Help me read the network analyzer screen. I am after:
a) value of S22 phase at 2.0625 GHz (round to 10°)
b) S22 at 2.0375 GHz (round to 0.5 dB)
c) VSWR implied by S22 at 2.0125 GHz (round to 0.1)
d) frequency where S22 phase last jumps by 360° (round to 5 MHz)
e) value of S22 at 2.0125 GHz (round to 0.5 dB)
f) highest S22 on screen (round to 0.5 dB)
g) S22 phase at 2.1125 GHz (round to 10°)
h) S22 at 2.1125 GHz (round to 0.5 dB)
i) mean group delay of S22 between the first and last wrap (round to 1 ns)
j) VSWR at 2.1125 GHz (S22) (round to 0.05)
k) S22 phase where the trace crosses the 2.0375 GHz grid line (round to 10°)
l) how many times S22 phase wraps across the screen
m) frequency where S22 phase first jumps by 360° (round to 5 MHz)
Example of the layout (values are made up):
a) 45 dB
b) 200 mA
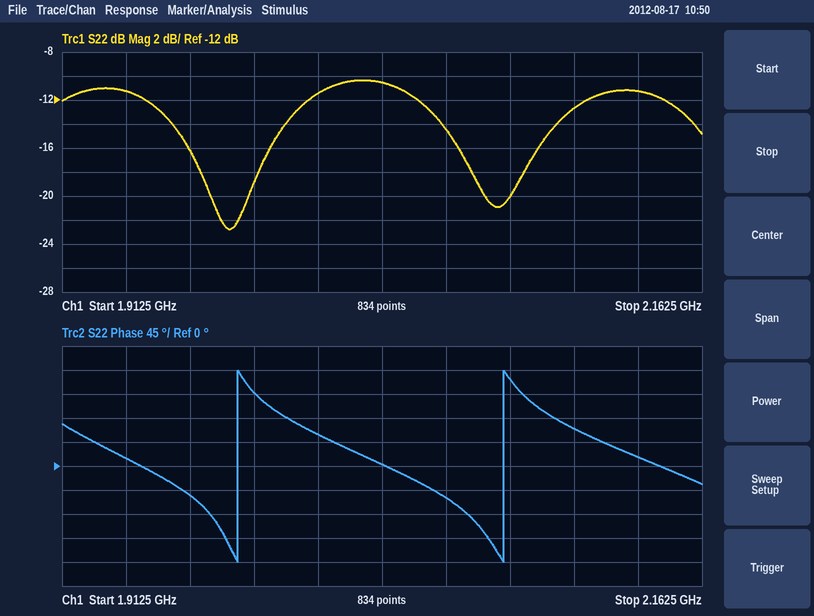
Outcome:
a) -60°
b) -10.5 dB
c) 1.7
d) 2.085 GHz
e) -11.5 dB
f) -10.5 dB
g) 70°
h) -12.5 dB
i) 10 ns
j) 1.60
k) 0°
l) 2
m) 1.980 GHz
